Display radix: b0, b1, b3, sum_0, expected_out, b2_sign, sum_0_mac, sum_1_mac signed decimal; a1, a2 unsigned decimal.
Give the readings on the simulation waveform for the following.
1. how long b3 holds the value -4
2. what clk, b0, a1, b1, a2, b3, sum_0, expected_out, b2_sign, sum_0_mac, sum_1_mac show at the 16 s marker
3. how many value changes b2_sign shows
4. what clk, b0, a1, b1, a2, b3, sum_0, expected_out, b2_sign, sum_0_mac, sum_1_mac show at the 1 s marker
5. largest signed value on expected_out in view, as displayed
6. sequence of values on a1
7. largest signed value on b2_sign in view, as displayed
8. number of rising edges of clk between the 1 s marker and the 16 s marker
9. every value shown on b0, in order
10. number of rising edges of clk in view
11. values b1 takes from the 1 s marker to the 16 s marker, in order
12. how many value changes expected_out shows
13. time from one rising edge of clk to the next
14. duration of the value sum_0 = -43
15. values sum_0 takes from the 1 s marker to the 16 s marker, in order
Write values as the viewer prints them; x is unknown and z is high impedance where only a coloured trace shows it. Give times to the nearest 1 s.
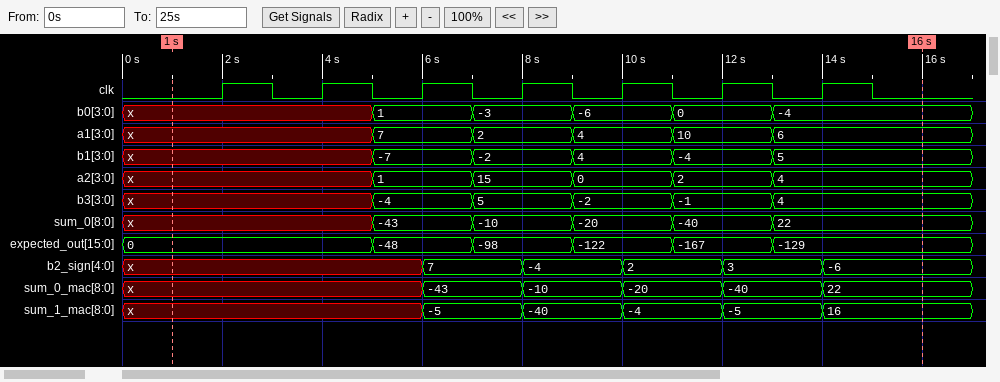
2 s
clk=0, b0=-4, a1=6, b1=5, a2=4, b3=4, sum_0=22, expected_out=-129, b2_sign=-6, sum_0_mac=22, sum_1_mac=16
5
clk=0, b0=x, a1=x, b1=x, a2=x, b3=x, sum_0=x, expected_out=0, b2_sign=x, sum_0_mac=x, sum_1_mac=x
0
x, 7, 2, 4, 10, 6
7
7
x, 1, -3, -6, 0, -4
7
x, -7, -2, 4, -4, 5
5
2 s
2 s
x, -43, -10, -20, -40, 22
